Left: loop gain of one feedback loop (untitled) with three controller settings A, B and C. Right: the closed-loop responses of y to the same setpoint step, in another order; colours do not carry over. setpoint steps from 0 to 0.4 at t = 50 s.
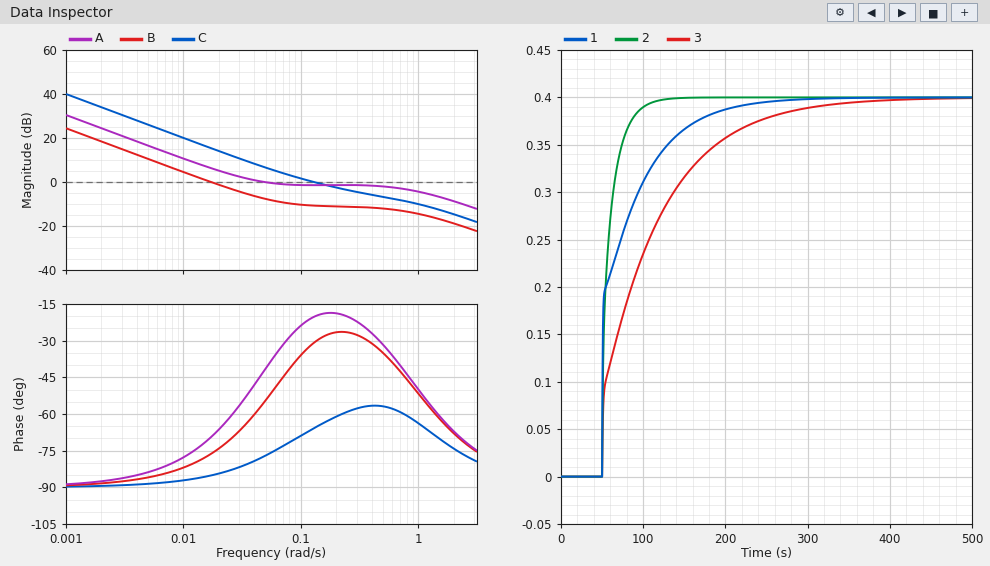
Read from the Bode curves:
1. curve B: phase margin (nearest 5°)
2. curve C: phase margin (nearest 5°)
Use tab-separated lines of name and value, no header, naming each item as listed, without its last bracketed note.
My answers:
curve B: phase margin	105°
curve C: phase margin	115°
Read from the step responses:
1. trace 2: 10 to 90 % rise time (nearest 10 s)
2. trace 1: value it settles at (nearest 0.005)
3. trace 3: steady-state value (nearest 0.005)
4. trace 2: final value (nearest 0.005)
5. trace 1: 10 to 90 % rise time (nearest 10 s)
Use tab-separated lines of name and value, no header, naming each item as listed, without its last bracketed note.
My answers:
trace 2: 10 to 90 % rise time	30 s
trace 1: value it settles at	0.400
trace 3: steady-state value	0.400
trace 2: final value	0.400
trace 1: 10 to 90 % rise time	90 s
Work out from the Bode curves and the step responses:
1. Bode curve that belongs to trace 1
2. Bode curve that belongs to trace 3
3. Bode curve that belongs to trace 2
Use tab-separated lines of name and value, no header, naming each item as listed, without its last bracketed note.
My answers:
Bode curve that belongs to trace 1	A
Bode curve that belongs to trace 3	B
Bode curve that belongs to trace 2	C
